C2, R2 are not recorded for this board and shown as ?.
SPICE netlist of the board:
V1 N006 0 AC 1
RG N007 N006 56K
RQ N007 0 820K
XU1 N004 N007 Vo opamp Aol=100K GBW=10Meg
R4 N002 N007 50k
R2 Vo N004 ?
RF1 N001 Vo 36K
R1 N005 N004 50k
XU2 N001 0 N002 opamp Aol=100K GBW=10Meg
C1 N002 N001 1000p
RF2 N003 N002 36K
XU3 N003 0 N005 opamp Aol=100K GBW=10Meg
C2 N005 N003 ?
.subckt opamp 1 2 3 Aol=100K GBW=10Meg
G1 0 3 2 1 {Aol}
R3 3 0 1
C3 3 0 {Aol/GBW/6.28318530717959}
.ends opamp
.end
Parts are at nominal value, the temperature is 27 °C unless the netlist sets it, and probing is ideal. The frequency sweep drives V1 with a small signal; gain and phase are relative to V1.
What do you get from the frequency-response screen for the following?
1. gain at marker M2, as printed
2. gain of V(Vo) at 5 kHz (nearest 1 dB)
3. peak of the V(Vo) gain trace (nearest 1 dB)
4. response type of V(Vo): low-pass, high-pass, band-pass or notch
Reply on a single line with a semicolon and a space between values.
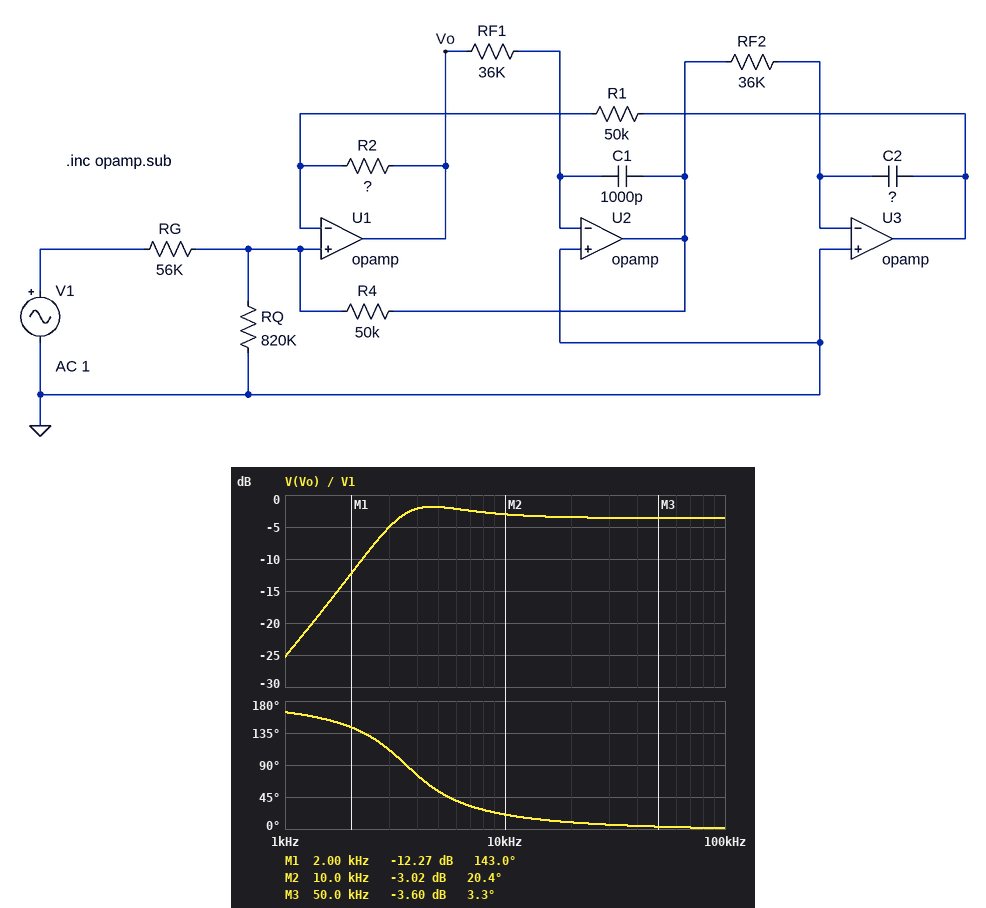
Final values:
-3.02 dB; -2 dB; -2 dB; high-pass
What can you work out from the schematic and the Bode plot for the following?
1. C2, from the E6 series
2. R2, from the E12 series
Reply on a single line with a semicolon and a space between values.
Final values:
680 pF; 22 kΩ
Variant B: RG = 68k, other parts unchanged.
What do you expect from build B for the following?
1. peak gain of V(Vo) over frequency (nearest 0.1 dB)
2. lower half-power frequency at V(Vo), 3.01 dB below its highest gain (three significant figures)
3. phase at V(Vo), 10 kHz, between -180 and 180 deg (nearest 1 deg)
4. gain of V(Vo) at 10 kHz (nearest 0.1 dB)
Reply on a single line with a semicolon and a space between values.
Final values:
-3.3 dB; 3.04 kHz; 22 deg; -4.1 dB
